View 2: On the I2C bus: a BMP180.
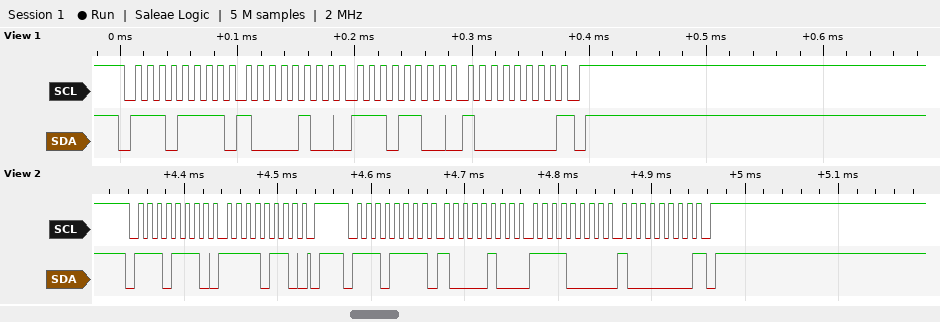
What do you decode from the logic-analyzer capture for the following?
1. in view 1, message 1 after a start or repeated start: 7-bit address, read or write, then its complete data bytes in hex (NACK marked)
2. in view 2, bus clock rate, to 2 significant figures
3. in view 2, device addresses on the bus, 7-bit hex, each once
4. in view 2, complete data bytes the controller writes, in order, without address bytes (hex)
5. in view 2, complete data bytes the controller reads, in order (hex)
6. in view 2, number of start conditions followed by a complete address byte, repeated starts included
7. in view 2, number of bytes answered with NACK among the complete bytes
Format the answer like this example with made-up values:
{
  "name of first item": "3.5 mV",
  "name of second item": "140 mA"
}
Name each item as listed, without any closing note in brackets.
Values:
{
  "in view 1, message 1 after a start or repeated start: 7-bit address, read or write, then its complete data bytes in hex": "0x77 read: 84 EC 80 NACK",
  "in view 2, bus clock rate, to 2 significant figures": "100 kHz",
  "in view 2, device addresses on the bus, 7-bit hex, each once": "0x77",
  "in view 2, complete data bytes the controller writes, in order, without address bytes": "F6",
  "in view 2, complete data bytes the controller reads, in order": "84 F0 80",
  "in view 2, number of start conditions followed by a complete address byte, repeated starts included": "2",
  "in view 2, number of bytes answered with NACK among the complete bytes": "1"
}
